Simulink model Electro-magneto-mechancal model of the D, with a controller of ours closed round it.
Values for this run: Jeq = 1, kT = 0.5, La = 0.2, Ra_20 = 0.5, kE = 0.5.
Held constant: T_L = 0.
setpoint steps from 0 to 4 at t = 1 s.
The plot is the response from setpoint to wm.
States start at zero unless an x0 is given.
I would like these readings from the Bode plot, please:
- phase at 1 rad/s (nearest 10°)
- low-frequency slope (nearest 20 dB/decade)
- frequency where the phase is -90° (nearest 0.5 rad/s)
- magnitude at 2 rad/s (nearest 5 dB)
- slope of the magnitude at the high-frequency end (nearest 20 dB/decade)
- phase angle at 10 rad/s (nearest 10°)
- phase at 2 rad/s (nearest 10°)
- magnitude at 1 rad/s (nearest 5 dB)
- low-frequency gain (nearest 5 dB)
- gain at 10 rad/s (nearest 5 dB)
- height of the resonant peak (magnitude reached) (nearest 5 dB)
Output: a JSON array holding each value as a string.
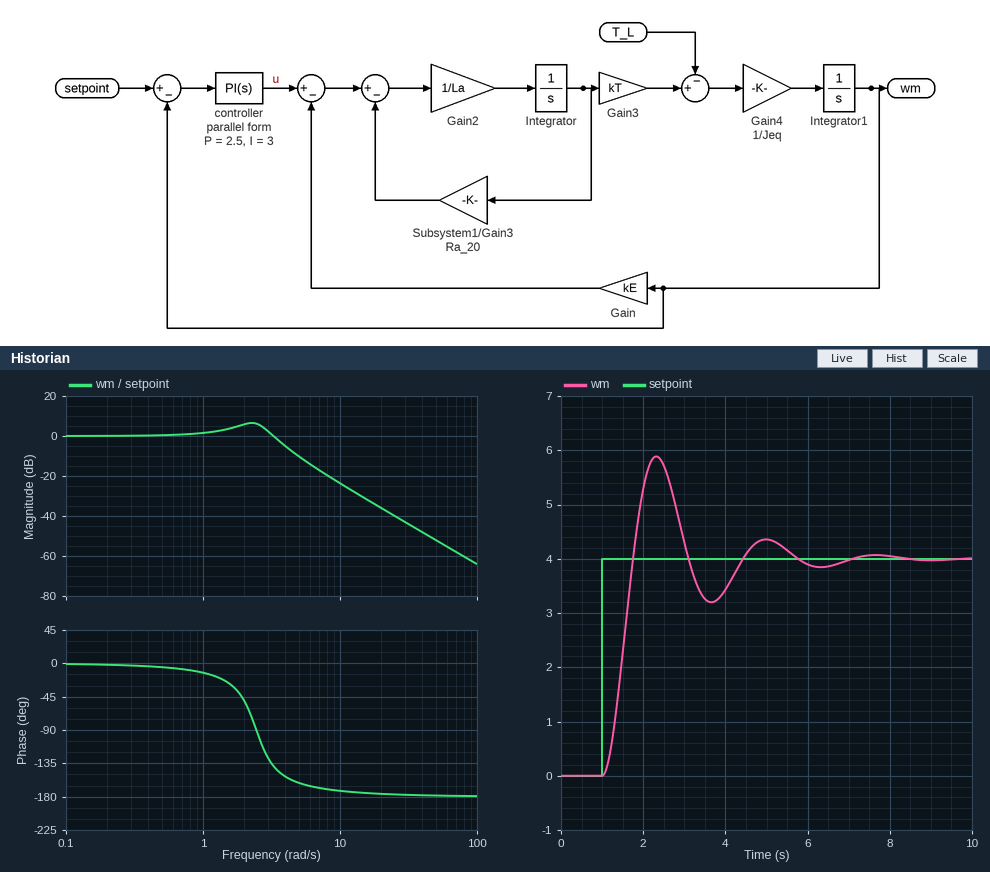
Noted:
["-10°", "0 dB/decade", "2.5 rad/s", "5 dB", "-40 dB/decade", "-170°", "-50°", "0 dB", "0 dB", "-25 dB", "5 dB"]
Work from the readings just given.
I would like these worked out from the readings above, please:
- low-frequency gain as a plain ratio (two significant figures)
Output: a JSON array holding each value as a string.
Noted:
["1.0"]
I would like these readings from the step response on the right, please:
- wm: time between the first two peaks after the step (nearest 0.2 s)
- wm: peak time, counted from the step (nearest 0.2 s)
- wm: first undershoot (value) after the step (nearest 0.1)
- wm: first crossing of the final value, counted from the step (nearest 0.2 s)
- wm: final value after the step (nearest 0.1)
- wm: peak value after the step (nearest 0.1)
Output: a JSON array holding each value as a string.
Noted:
["2.6 s", "1.4 s", "3.2", "0.8 s", "4.0", "5.9"]
